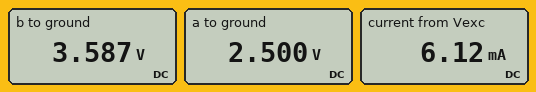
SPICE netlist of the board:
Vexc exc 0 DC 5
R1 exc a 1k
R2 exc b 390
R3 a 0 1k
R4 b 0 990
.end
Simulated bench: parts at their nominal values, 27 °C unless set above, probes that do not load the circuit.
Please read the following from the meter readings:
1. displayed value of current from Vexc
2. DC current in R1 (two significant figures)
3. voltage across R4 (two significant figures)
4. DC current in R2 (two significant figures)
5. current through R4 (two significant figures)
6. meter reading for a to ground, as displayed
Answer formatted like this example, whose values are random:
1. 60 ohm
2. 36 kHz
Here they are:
1. 6.12 mA
2. 2.5 mA
3. 3.6 V
4. 3.6 mA
5. 3.6 mA
6. 2.500 V
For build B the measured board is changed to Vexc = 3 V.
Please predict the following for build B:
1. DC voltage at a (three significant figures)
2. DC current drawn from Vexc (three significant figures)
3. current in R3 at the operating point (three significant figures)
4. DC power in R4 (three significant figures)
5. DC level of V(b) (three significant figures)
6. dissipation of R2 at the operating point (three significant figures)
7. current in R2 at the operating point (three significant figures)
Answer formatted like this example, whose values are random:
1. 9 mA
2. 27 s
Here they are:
1. 1.50 V
2. 3.67 mA
3. 1.50 mA
4. 4.68 mW
5. 2.15 V
6. 1.84 mW
7. 2.17 mA
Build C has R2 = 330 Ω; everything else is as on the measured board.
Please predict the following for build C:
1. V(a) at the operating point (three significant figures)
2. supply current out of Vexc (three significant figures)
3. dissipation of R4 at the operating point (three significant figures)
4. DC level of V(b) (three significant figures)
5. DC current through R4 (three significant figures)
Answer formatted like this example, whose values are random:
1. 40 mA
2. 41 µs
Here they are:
1. 2.50 V
2. 6.29 mA
3. 14.2 mW
4. 3.75 V
5. 3.79 mA
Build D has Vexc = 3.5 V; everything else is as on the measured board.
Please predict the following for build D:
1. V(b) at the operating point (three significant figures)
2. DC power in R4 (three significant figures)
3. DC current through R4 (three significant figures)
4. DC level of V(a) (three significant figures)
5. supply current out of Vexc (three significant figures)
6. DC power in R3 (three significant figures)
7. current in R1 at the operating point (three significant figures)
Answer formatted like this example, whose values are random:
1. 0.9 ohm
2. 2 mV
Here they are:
1. 2.51 V
2. 6.37 mW
3. 2.54 mA
4. 1.75 V
5. 4.29 mA
6. 3.06 mW
7. 1.75 mA
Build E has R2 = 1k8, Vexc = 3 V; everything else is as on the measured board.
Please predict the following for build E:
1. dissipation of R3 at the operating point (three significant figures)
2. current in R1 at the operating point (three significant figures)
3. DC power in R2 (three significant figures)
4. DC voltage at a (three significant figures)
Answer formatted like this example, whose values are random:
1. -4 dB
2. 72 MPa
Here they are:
1. 2.25 mW
2. 1.50 mA
3. 2.08 mW
4. 1.50 V
